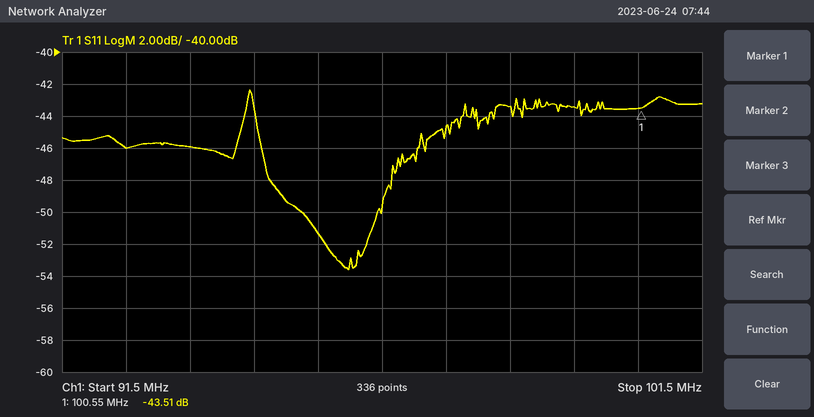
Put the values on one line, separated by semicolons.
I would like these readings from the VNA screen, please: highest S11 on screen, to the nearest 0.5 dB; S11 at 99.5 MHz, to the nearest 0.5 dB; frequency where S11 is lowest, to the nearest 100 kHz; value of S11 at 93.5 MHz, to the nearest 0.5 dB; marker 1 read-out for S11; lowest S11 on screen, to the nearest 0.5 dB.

-42.5 dB; -43.5 dB; 96.0 MHz; -46.0 dB; -43.51 dB; -53.5 dB
